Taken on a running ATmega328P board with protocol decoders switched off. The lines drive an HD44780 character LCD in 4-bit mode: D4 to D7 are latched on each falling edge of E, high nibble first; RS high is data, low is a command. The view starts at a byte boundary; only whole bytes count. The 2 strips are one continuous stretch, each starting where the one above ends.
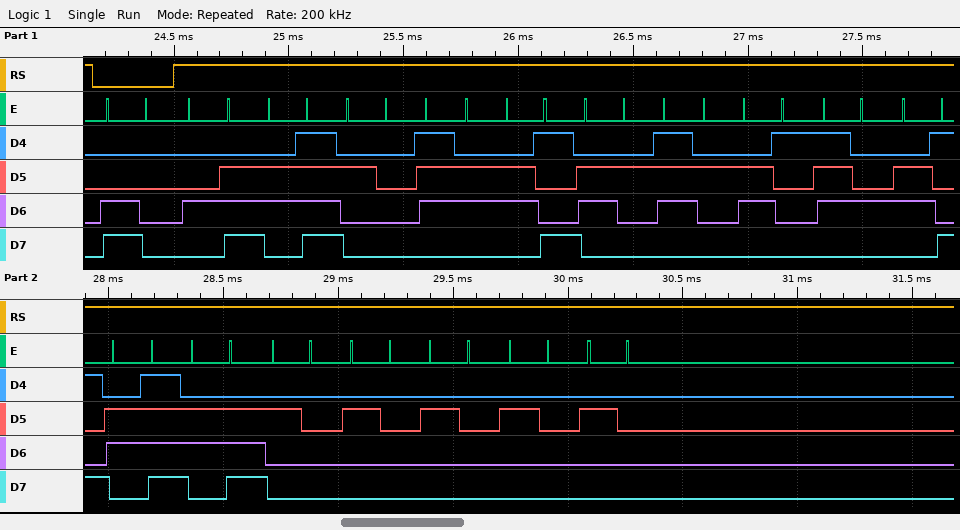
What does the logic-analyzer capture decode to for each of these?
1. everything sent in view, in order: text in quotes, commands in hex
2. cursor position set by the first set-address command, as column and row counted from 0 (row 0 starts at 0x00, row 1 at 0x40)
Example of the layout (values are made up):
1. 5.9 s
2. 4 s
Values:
1. 0xC0 "No vibration     "
2. column 0, row 1
